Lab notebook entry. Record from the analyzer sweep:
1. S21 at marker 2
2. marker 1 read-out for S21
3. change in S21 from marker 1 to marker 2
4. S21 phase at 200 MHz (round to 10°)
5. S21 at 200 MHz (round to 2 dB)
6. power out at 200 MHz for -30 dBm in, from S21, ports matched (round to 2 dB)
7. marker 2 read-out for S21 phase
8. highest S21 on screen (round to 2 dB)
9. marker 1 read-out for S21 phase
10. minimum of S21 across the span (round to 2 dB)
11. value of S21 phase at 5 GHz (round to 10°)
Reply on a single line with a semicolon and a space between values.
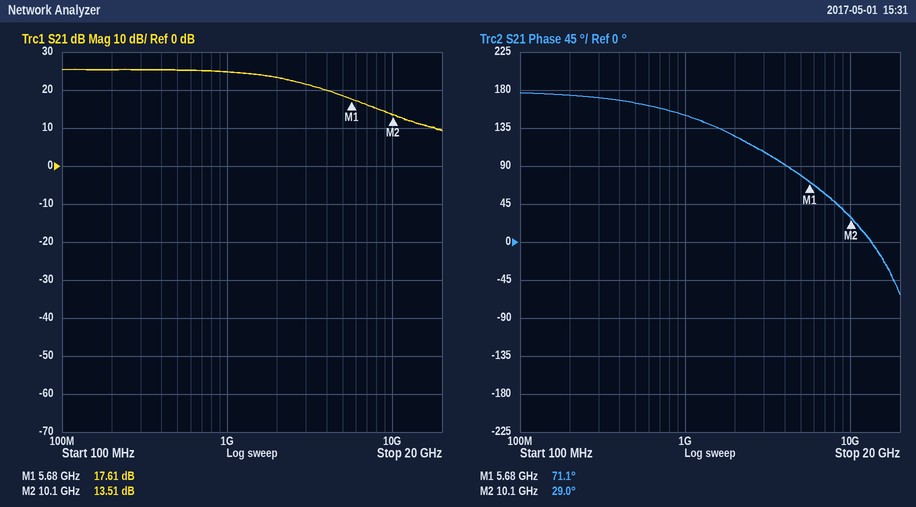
13.51 dB; 17.61 dB; -4.10 dB; 170°; 26 dB; -4 dBm; 29.0°; 26 dB; 71.1°; 10 dB; 80°
